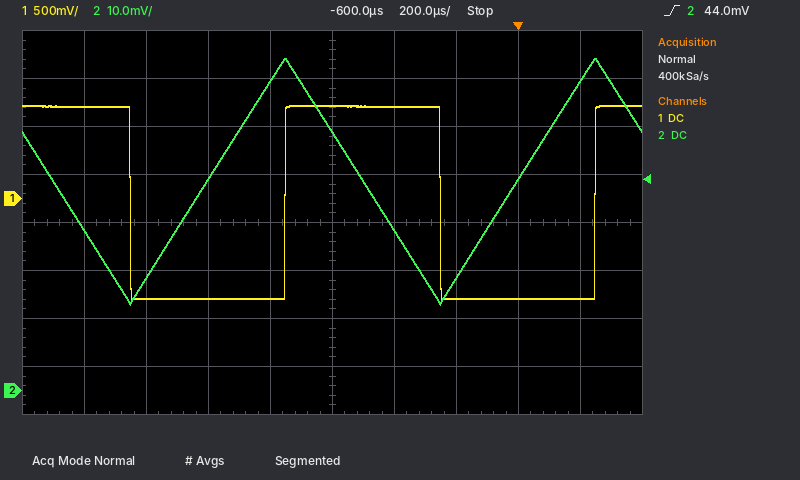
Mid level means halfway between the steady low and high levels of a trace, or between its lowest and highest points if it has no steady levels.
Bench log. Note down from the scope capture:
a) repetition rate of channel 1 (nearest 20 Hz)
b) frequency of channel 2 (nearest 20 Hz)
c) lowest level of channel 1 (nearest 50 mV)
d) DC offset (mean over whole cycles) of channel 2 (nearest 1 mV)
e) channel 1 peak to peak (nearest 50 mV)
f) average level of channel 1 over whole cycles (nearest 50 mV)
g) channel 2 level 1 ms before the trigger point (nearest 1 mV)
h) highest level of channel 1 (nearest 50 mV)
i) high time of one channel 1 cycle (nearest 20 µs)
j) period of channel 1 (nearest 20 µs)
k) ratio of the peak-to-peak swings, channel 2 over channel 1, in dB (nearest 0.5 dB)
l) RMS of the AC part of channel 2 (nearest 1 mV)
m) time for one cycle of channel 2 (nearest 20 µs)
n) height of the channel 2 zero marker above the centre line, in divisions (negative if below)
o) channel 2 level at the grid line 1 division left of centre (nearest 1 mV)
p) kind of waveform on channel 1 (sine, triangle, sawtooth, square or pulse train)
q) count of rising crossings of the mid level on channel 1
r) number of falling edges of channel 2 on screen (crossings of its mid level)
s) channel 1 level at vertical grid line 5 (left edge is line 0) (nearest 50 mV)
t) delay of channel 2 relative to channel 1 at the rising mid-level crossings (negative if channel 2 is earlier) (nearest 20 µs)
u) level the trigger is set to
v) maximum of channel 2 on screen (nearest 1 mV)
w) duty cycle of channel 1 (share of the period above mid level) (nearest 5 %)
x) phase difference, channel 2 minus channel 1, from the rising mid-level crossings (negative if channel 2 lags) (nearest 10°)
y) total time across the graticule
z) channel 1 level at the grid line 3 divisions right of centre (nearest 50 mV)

1.00 kHz
1.00 kHz
-1.05 V
44 mV
2.00 V
-50 mV
44 mV
950 mV
500 µs
1.00 ms
-32.0 dB
15 mV
1.00 ms
-3.5 div
64 mV
square
2
2
950 mV
-260 µs
44.0 mV
69 mV
50 %
+90°
2 ms
-1.05 V
